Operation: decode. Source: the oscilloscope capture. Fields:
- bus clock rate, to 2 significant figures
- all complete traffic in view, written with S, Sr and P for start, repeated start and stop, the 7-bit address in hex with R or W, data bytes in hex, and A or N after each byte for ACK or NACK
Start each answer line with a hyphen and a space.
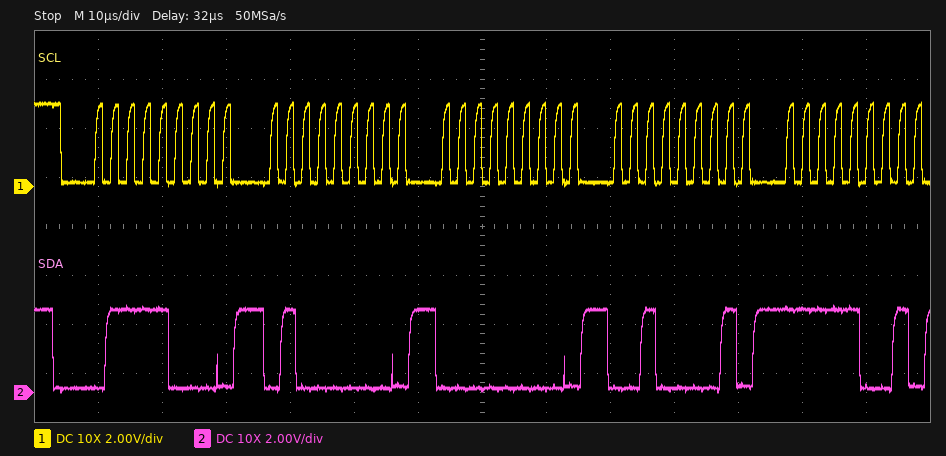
- 400 kHz
- S 3CW A 40 A 00 A 21 A F9 A
